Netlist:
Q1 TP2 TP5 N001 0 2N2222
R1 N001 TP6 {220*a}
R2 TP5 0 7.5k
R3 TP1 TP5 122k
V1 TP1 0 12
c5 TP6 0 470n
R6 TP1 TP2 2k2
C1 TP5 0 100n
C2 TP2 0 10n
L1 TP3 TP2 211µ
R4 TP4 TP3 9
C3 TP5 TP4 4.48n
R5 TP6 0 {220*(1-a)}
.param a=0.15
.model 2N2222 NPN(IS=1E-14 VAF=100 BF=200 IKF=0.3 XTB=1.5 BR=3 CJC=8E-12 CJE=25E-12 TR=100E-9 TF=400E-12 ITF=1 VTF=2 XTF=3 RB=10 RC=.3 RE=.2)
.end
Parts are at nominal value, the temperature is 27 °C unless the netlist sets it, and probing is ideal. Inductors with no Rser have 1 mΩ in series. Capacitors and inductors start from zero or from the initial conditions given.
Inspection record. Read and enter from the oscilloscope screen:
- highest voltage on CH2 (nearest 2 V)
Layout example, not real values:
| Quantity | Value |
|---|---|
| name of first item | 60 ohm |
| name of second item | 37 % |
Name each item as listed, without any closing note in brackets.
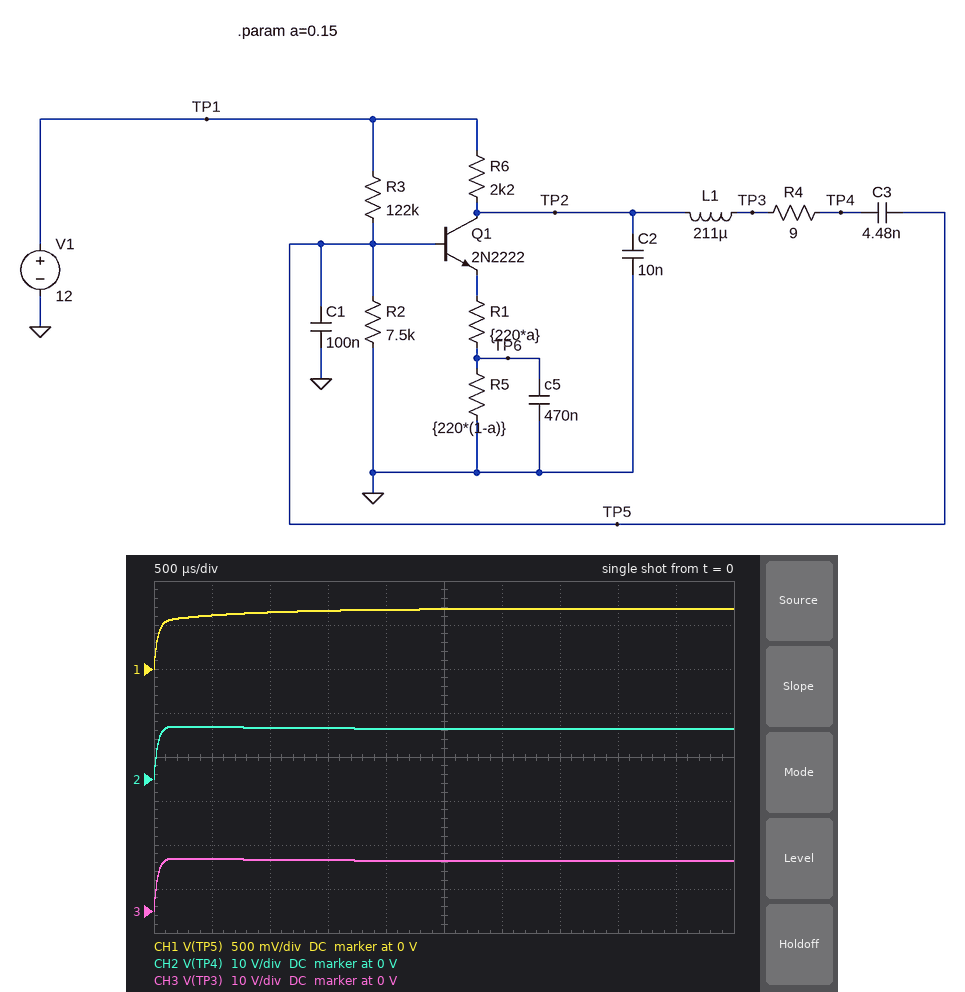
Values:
| Quantity | Value |
|---|---|
| highest voltage on CH2 | 12 V |
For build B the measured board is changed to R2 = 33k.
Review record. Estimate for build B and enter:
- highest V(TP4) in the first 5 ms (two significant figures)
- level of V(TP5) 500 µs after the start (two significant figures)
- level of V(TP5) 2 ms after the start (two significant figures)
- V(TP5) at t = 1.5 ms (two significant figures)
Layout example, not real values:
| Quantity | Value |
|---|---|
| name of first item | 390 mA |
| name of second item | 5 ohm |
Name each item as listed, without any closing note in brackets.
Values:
| Quantity | Value |
|---|---|
| highest V(TP4) in the first 5 ms | 12 V |
| level of V(TP5) 500 µs after the start | 790 mV |
| level of V(TP5) 2 ms after the start | 1.3 V |
| V(TP5) at t = 1.5 ms | 1.2 V |
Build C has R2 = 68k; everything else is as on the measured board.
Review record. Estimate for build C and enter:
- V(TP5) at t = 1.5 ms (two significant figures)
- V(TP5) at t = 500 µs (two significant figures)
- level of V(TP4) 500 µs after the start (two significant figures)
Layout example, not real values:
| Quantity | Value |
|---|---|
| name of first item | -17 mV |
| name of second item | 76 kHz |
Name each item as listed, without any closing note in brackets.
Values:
| Quantity | Value |
|---|---|
| V(TP5) at t = 1.5 ms | 1.3 V |
| V(TP5) at t = 500 µs | 820 mV |
| level of V(TP4) 500 µs after the start | 10 V |
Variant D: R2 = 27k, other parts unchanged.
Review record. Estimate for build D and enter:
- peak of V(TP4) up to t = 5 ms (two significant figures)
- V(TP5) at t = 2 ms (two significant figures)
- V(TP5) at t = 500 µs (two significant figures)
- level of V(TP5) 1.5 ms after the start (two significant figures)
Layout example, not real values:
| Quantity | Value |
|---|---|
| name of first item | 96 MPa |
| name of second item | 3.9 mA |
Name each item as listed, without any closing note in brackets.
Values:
| Quantity | Value |
|---|---|
| peak of V(TP4) up to t = 5 ms | 12 V |
| V(TP5) at t = 2 ms | 1.2 V |
| V(TP5) at t = 500 µs | 780 mV |
| level of V(TP5) 1.5 ms after the start | 1.1 V |
